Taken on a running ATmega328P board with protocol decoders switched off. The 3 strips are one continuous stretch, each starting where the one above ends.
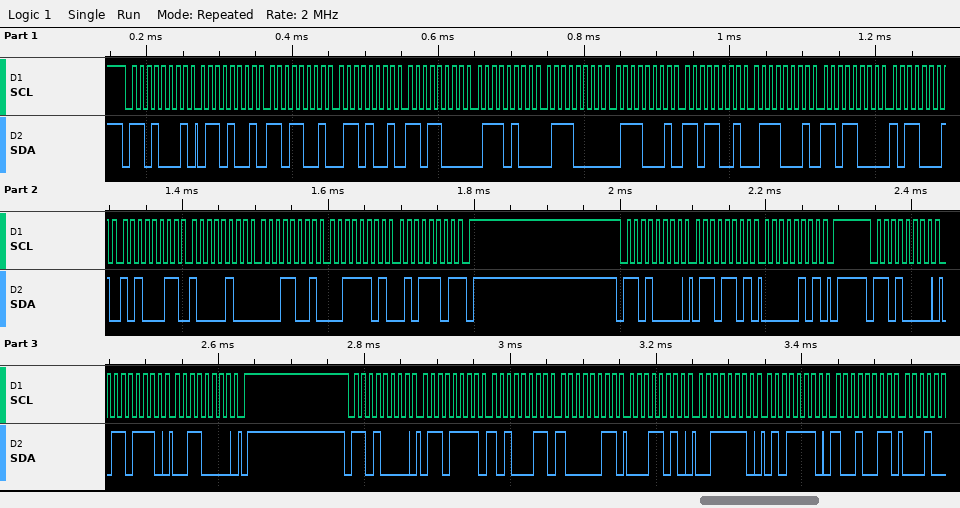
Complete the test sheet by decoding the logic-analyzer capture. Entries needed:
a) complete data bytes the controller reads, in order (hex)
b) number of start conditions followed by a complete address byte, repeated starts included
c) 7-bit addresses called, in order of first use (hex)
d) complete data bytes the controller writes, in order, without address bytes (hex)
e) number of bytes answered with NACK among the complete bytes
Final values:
69 D9 69 D8 74 70 71 D9 71 D8 B1 A3 84 19 3D 5D
4
0x68
6D 05 6E 30 6F A3 83 1A 3E 5E 93
1
